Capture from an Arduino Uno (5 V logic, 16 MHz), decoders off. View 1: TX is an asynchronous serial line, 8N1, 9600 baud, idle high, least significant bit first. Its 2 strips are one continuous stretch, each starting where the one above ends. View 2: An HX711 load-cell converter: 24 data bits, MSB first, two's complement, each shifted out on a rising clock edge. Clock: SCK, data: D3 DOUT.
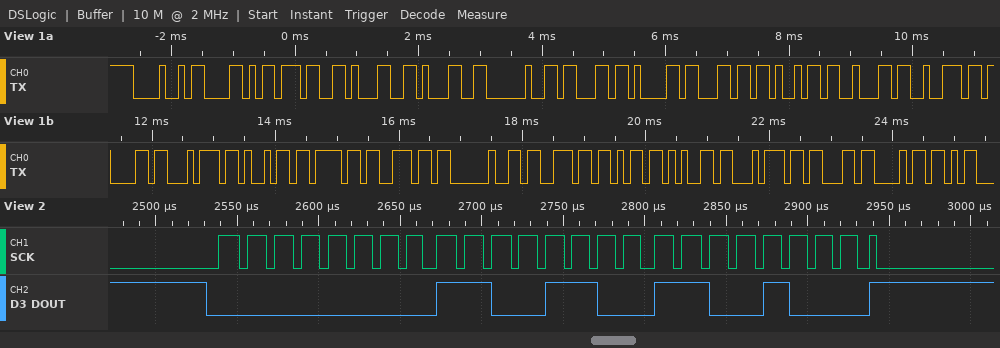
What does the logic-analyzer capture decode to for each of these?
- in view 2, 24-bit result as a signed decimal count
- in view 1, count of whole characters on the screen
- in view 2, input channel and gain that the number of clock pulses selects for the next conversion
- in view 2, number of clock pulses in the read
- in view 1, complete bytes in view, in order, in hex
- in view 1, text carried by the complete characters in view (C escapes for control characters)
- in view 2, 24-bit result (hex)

52424
24
channel A, gain 128
25
0x48 0x58 0x37 0x31 0x31 0x20 0x63 0x61 0x6C 0x69 0x62 0x72 0x61 0x74 0x69 0x6F 0x6E 0x20 0x73 0x6B 0x65 0x74 0x63 0x68
"HX711 calibration sketch"
0x00CCC8
